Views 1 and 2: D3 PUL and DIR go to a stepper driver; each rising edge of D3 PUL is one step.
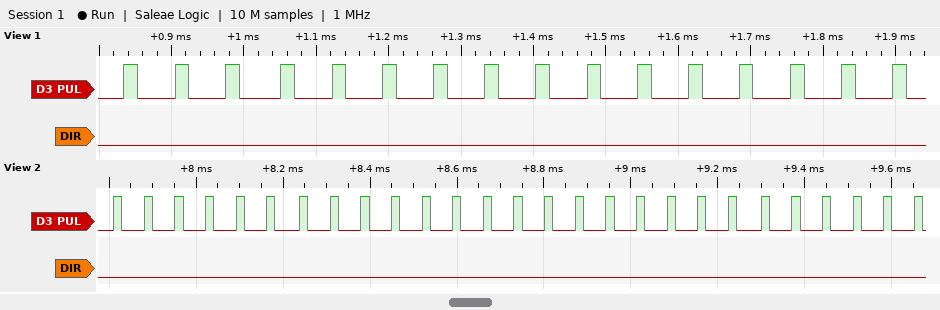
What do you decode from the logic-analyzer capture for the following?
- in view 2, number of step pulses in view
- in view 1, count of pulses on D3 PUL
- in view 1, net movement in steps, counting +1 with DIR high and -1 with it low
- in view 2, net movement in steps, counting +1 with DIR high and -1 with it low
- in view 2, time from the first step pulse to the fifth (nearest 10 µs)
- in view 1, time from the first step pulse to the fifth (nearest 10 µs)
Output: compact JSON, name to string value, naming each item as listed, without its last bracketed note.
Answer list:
{"in view 2, number of step pulses in view": "27", "in view 1, count of pulses on D3 PUL": "16", "in view 1, net movement in steps, counting +1 with DIR high and -1 with it low": "-16", "in view 2, net movement in steps, counting +1 with DIR high and -1 with it low": "-27", "in view 2, time from the first step pulse to the fifth": "280 µs", "in view 1, time from the first step pulse to the fifth": "290 µs"}
